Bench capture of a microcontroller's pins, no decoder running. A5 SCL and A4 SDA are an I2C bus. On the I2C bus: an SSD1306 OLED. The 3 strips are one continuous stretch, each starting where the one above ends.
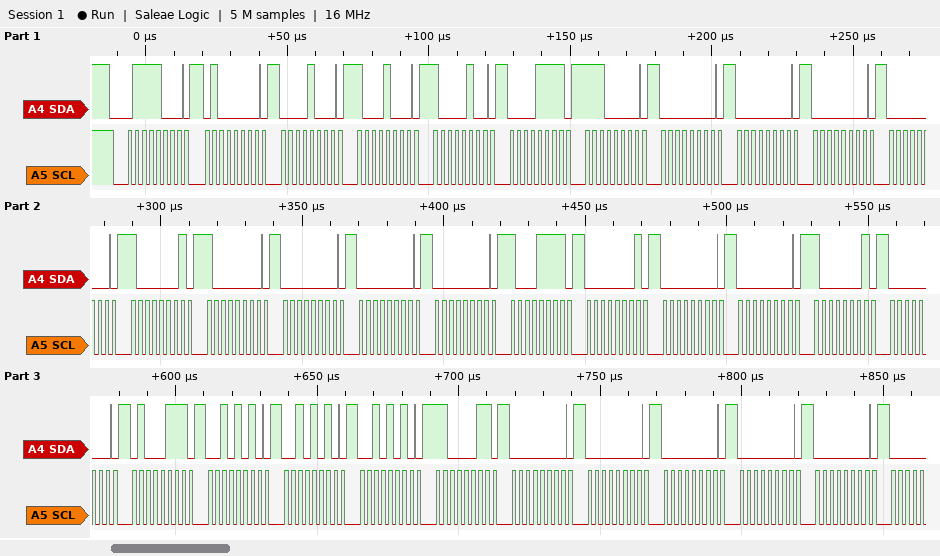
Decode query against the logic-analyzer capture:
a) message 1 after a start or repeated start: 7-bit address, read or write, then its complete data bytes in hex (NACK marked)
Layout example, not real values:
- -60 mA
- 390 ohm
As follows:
- 0x3C write: 40 08 88 84 0F E0 00 00 00 00 81 80 00 00 00 8F 01 00 00 81 00 47 2A 2A 2A C3 00 00 00 00 00
